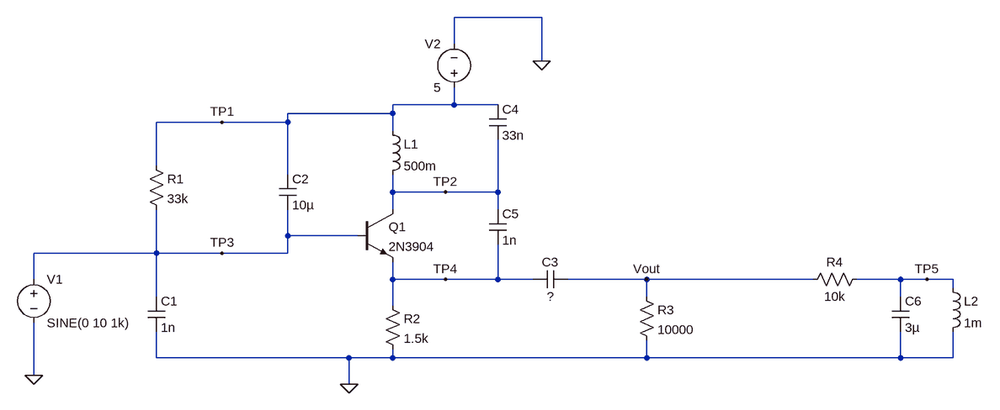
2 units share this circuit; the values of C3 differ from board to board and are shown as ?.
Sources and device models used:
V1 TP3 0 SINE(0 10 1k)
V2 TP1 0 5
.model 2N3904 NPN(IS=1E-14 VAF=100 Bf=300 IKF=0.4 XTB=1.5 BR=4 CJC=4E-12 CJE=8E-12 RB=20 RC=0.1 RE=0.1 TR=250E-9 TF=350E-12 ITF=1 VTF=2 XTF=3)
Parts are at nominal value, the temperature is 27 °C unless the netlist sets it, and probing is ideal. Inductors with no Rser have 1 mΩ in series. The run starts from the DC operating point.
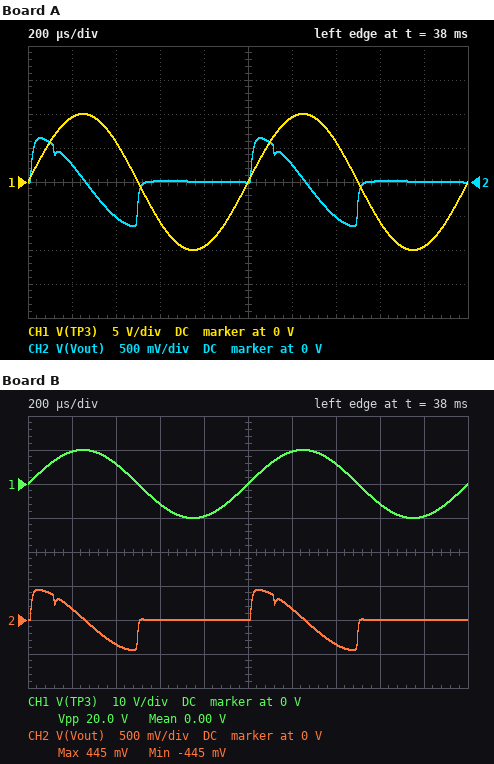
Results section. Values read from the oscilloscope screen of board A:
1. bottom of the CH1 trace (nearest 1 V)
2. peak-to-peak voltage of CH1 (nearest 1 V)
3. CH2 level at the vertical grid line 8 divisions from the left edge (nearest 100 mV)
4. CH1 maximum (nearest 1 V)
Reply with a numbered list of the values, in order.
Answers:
1. -10 V
2. 20 V
3. 0 V
4. 10 V
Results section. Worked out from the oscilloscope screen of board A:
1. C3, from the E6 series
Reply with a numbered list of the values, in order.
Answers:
1. 2.2 nF
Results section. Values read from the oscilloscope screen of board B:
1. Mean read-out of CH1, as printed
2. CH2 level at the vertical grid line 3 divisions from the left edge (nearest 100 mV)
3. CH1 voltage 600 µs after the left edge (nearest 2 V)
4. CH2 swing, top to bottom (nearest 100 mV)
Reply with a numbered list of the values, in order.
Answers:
1. 0.00 V
2. 0 V
3. -6 V
4. 900 mV
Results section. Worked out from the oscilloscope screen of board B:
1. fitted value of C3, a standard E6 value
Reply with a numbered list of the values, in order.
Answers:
1. 1.5 nF
